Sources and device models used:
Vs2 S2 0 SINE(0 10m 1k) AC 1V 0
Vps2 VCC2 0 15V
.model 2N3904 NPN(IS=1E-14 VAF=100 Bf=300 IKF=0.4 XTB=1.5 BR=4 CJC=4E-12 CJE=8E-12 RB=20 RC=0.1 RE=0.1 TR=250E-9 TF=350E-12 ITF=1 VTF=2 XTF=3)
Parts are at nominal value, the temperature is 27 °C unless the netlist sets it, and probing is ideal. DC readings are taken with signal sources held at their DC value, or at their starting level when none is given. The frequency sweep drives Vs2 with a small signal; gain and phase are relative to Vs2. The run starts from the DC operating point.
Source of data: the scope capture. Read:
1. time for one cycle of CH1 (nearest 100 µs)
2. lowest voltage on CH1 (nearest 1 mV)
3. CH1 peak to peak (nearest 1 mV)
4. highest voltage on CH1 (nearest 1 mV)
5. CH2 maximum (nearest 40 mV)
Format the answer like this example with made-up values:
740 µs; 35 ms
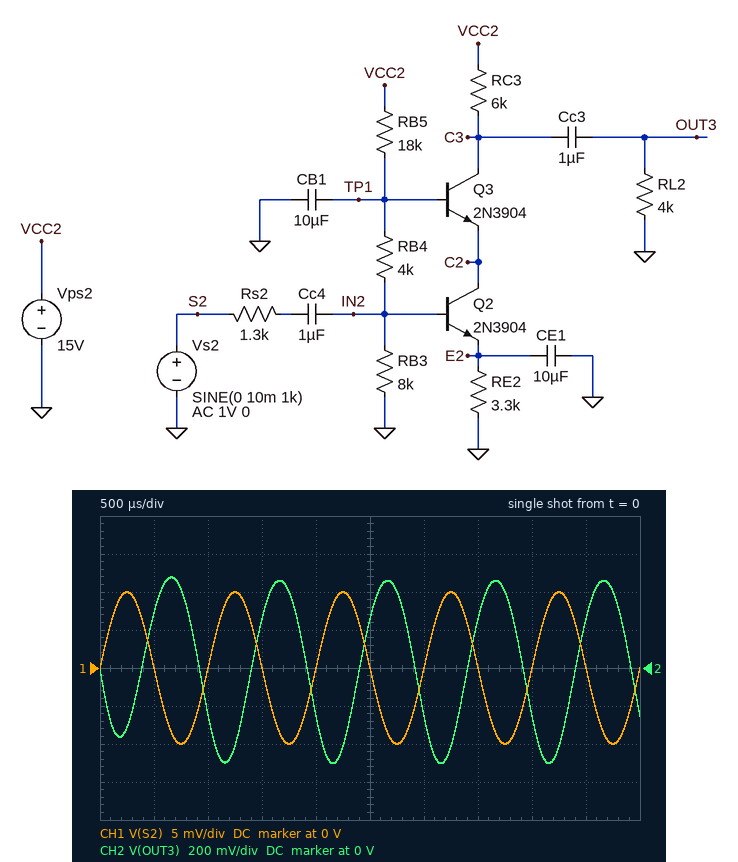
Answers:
1.0 ms; -10 mV; 20 mV; 10 mV; 480 mV
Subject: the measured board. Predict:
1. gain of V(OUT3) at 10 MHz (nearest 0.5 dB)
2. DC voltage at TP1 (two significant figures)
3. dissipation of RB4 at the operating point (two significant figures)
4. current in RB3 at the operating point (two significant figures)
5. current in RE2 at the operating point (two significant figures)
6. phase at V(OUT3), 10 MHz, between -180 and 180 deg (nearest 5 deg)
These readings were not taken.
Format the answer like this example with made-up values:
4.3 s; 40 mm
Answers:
29.0 dB; 6.0 V; 1.0 mW; 500 µA; 1.0 mA; 100 deg
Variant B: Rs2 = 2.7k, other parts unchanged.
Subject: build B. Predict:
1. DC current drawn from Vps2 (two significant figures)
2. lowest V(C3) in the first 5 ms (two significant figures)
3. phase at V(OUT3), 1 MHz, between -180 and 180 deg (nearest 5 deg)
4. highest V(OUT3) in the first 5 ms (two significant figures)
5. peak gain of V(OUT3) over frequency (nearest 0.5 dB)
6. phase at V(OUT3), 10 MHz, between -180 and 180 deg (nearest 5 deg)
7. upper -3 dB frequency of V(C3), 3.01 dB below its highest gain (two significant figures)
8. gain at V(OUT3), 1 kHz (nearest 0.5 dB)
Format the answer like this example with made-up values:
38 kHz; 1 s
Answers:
1.5 mA; 8.7 V; 165 deg; 350 mV; 32.0 dB; 90 deg; 4.3 MHz; 30.5 dB
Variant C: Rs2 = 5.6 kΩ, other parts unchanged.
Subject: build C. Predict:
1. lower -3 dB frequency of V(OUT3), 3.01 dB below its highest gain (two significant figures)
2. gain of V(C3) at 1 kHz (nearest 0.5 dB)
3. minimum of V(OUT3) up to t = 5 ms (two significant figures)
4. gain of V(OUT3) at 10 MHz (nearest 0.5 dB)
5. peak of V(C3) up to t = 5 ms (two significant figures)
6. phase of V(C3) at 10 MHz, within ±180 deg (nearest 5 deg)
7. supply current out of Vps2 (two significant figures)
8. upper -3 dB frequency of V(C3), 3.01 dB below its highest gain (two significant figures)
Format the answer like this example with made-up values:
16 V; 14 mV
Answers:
510 Hz; 26.5 dB; -220 mV; 17.0 dB; 9.2 V; 85 deg; 1.5 mA; 3.4 MHz
